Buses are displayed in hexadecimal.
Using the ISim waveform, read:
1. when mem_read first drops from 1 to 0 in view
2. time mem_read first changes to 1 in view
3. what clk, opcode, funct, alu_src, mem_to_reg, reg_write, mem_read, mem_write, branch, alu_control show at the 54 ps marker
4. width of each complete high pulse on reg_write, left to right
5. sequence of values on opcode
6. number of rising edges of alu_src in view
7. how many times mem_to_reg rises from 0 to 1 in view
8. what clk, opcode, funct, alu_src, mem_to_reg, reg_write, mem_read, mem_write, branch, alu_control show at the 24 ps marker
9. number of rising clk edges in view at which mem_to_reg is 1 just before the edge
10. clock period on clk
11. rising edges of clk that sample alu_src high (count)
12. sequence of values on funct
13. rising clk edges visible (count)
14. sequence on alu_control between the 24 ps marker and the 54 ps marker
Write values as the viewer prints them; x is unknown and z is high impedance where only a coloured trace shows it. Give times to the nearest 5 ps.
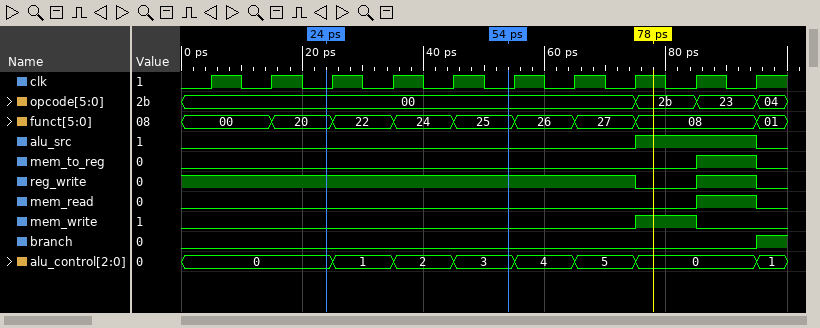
95 ps
85 ps
clk=0, opcode=00, funct=25, alu_src=0, mem_to_reg=0, reg_write=1, mem_read=0, mem_write=0, branch=0, alu_control=3
10 ps
00, 2b, 23, 04
1
1
clk=0, opcode=00, funct=20, alu_src=0, mem_to_reg=0, reg_write=1, mem_read=0, mem_write=0, branch=0, alu_control=0
1
10 ps
2
00, 20, 22, 24, 25, 26, 27, 08, 01
10
0, 1, 2, 3
